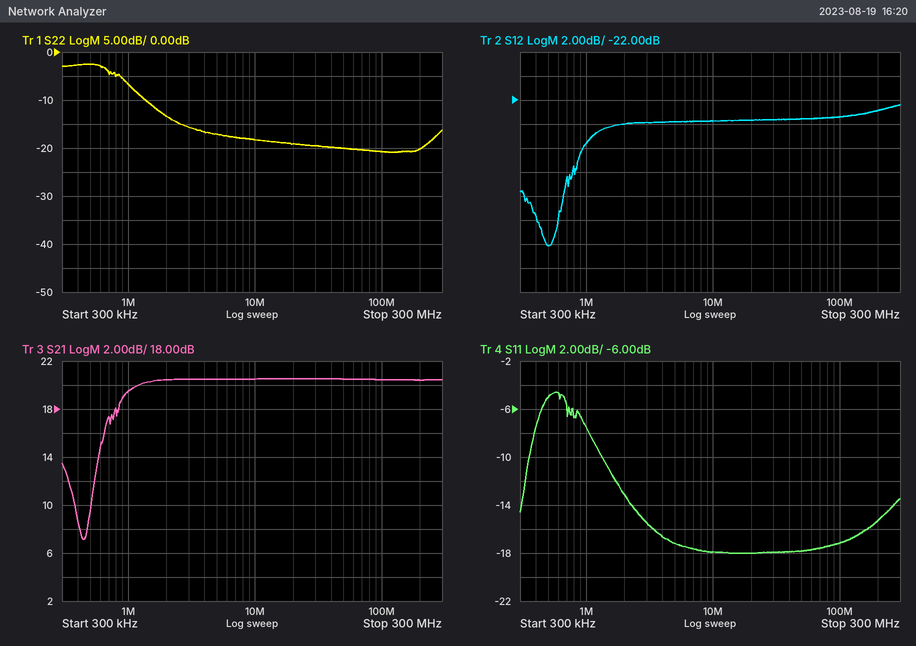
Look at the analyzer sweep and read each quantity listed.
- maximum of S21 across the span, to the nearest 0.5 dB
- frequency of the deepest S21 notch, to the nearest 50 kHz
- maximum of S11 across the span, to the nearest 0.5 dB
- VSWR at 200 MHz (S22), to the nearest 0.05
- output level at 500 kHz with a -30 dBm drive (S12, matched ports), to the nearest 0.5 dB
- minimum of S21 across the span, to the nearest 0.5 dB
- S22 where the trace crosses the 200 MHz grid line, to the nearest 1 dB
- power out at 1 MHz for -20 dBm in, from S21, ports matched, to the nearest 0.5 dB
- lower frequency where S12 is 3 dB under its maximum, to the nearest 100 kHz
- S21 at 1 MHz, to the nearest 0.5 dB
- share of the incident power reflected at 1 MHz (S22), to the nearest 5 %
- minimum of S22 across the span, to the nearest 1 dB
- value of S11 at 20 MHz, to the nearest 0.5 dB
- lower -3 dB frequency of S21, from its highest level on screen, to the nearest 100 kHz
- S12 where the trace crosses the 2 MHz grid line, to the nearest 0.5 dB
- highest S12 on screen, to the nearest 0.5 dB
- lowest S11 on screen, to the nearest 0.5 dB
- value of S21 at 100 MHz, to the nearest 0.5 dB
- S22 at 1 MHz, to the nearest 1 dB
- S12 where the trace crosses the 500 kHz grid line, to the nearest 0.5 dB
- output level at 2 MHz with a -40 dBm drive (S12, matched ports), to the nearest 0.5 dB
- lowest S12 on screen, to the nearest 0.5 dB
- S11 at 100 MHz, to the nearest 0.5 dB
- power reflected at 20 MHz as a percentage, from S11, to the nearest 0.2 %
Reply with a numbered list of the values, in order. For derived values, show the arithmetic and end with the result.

1. 20.5 dB
2. 450 kHz
3. -4.5 dB
4. |Γ| = 10^(-20/20) = 0.1000; VSWR = (1 + 0.1000)/(1 − 0.1000) ≈ 1.22, so 1.20 to the nearest 0.05
5. -30 dBm + (-34.0 dB) = -64.0 dBm
6. 7.0 dB
7. -20 dB
8. -20 dBm + (19.5 dB) = -0.5 dBm
9. 1.0 MHz
10. 19.5 dB
11. 10^(-7/10) ≈ 20 %
12. -21 dB
13. -18.0 dB
14. 800 kHz
15. -24.0 dB
16. -22.5 dB
17. -18.0 dB
18. 20.5 dB
19. -7 dB
20. -34.0 dB
21. -40 dBm + (-24.0 dB) = -64.0 dBm
22. -34.0 dB
23. -17.0 dB
24. 10^(-18/10) ≈ 1.6 %
